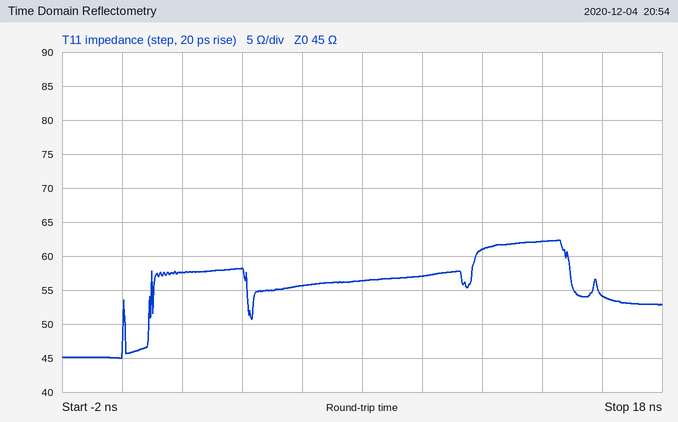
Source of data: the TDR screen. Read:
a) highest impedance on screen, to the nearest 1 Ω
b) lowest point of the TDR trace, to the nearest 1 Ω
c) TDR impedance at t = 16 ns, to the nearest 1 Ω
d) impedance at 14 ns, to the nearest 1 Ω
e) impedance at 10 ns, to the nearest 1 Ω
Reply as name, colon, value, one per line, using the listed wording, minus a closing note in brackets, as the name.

highest impedance on screen, to the nearest 1 Ω: 62 Ω
lowest point of the TDR trace, to the nearest 1 Ω: 45 Ω
TDR impedance at t = 16 ns, to the nearest 1 Ω: 54 Ω
impedance at 14 ns, to the nearest 1 Ω: 62 Ω
impedance at 10 ns, to the nearest 1 Ω: 57 Ω
